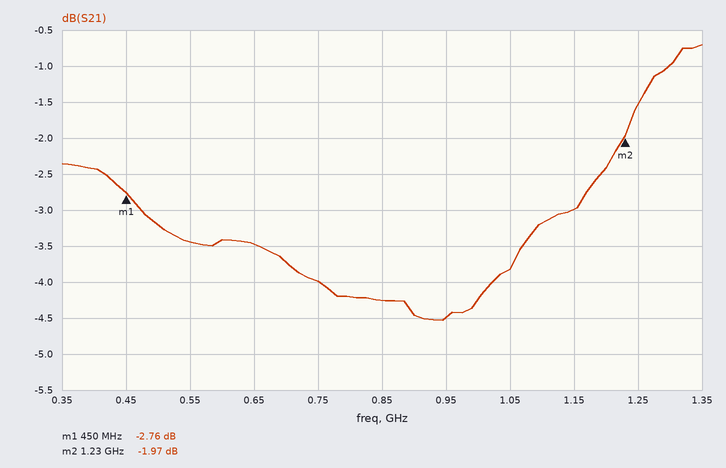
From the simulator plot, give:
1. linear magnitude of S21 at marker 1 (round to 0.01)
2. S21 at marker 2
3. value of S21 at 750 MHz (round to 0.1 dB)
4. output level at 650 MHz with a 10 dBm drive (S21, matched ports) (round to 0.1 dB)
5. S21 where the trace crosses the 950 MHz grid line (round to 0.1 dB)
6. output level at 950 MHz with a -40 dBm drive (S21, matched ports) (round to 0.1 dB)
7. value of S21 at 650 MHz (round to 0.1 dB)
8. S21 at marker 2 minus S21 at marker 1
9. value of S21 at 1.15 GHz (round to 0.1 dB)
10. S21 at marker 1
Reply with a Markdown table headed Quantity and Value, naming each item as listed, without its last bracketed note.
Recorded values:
| Quantity | Value |
|---|---|
| linear magnitude of S21 at marker 1 | 0.73 |
| S21 at marker 2 | -1.97 dB |
| value of S21 at 750 MHz | -4.0 dB |
| output level at 650 MHz with a 10 dBm drive (S21, matched ports) | 6.5 dBm |
| S21 where the trace crosses the 950 MHz grid line | -4.5 dB |
| output level at 950 MHz with a -40 dBm drive (S21, matched ports) | -44.5 dBm |
| value of S21 at 650 MHz | -3.5 dB |
| S21 at marker 2 minus S21 at marker 1 | 0.79 dB |
| value of S21 at 1.15 GHz | -3.0 dB |
| S21 at marker 1 | -2.76 dB |
